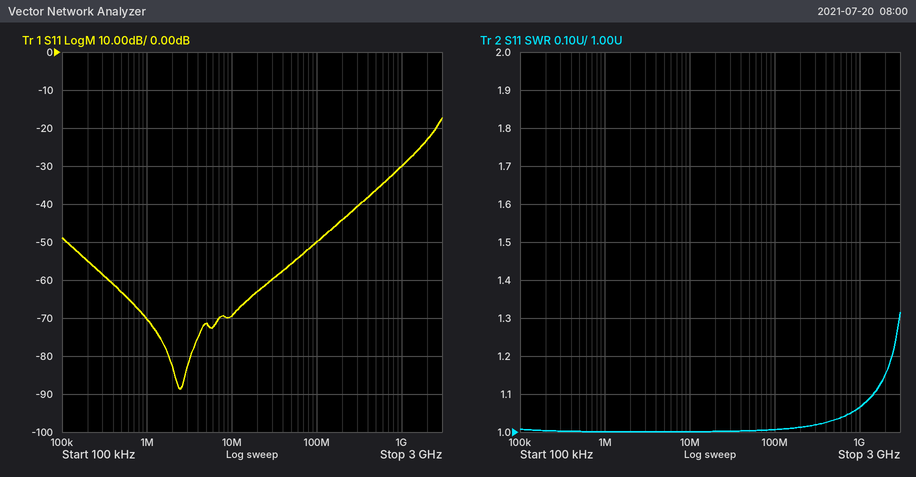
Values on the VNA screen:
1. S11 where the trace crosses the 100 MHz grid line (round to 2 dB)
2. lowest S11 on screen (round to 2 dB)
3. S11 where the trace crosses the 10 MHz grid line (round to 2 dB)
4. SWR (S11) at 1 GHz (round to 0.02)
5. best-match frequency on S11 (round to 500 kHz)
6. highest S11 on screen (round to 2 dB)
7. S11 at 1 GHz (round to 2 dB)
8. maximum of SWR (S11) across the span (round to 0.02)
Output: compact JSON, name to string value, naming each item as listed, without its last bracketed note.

{"S11 where the trace crosses the 100 MHz grid line": "-50 dB", "lowest S11 on screen": "-88 dB", "S11 where the trace crosses the 10 MHz grid line": "-70 dB", "SWR (S11) at 1 GHz": "1.06", "best-match frequency on S11": "2.5 MHz", "highest S11 on screen": "-18 dB", "S11 at 1 GHz": "-30 dB", "maximum of SWR (S11) across the span": "1.32"}
